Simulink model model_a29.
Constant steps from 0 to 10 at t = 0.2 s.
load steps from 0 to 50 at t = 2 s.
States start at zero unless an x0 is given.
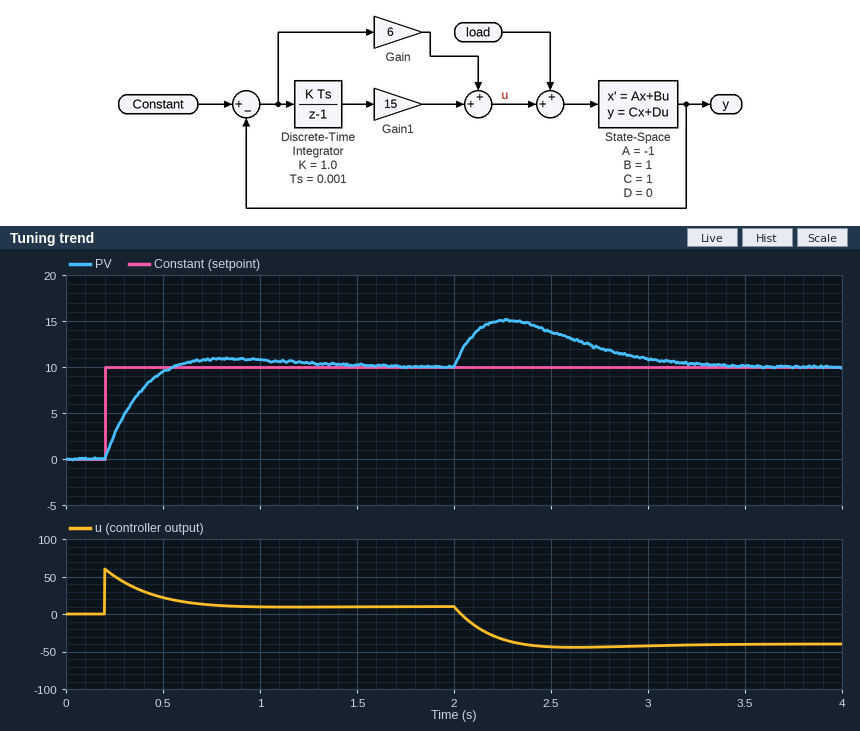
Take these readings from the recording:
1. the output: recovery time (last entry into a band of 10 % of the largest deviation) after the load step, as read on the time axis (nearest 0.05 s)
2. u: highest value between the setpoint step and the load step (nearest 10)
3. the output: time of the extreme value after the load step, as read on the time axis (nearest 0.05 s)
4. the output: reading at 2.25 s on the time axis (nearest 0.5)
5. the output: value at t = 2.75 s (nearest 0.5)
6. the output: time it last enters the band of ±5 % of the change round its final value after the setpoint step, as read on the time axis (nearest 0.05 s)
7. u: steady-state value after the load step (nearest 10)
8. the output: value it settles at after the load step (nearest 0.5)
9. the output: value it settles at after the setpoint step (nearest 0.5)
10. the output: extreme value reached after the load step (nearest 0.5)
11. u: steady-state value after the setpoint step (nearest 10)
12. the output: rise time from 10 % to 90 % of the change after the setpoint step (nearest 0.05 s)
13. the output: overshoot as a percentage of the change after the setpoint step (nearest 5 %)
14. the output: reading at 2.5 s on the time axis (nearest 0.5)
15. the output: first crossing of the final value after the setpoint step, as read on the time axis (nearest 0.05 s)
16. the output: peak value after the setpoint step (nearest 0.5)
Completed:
3.15 s
60
2.25 s
15.0
12.0
1.20 s
-40
10.0
10.0
15.0
10
0.25 s
10 %
14.0
0.55 s
11.0
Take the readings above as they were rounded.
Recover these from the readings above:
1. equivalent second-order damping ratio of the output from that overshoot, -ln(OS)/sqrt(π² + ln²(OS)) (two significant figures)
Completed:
0.59
